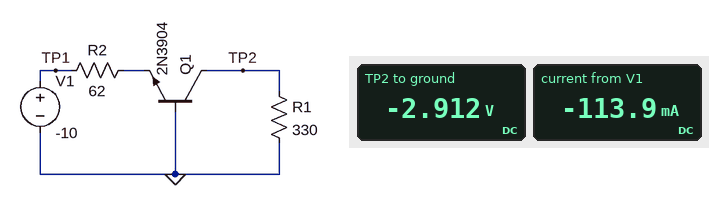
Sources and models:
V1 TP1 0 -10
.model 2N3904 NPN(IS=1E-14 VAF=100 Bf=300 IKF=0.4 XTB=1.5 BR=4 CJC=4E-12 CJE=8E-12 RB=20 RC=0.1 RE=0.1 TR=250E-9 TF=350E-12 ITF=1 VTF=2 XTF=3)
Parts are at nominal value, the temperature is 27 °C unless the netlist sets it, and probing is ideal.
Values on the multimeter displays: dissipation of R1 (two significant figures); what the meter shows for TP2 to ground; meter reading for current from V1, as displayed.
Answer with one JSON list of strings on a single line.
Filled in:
["26 mW", "-2.912 V", "-113.9 mA"]
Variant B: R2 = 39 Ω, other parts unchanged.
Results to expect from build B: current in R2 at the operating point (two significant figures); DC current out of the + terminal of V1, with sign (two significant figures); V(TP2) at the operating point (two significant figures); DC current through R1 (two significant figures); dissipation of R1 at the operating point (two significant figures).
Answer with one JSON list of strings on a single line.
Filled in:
["160 mA", "-160 mA", "-3.8 V", "11 mA", "43 mW"]
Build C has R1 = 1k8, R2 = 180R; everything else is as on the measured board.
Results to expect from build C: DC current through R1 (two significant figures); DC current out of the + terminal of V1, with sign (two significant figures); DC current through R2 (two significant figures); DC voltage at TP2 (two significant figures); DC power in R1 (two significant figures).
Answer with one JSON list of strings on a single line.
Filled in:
["940 µA", "-46 mA", "46 mA", "-1.7 V", "1.6 mW"]
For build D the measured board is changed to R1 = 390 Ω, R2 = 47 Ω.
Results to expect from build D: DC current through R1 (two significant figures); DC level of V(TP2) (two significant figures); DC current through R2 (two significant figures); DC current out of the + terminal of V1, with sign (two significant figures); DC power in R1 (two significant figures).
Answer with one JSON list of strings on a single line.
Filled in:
["8.8 mA", "-3.4 V", "140 mA", "-140 mA", "30 mW"]
